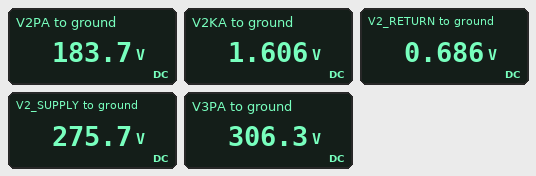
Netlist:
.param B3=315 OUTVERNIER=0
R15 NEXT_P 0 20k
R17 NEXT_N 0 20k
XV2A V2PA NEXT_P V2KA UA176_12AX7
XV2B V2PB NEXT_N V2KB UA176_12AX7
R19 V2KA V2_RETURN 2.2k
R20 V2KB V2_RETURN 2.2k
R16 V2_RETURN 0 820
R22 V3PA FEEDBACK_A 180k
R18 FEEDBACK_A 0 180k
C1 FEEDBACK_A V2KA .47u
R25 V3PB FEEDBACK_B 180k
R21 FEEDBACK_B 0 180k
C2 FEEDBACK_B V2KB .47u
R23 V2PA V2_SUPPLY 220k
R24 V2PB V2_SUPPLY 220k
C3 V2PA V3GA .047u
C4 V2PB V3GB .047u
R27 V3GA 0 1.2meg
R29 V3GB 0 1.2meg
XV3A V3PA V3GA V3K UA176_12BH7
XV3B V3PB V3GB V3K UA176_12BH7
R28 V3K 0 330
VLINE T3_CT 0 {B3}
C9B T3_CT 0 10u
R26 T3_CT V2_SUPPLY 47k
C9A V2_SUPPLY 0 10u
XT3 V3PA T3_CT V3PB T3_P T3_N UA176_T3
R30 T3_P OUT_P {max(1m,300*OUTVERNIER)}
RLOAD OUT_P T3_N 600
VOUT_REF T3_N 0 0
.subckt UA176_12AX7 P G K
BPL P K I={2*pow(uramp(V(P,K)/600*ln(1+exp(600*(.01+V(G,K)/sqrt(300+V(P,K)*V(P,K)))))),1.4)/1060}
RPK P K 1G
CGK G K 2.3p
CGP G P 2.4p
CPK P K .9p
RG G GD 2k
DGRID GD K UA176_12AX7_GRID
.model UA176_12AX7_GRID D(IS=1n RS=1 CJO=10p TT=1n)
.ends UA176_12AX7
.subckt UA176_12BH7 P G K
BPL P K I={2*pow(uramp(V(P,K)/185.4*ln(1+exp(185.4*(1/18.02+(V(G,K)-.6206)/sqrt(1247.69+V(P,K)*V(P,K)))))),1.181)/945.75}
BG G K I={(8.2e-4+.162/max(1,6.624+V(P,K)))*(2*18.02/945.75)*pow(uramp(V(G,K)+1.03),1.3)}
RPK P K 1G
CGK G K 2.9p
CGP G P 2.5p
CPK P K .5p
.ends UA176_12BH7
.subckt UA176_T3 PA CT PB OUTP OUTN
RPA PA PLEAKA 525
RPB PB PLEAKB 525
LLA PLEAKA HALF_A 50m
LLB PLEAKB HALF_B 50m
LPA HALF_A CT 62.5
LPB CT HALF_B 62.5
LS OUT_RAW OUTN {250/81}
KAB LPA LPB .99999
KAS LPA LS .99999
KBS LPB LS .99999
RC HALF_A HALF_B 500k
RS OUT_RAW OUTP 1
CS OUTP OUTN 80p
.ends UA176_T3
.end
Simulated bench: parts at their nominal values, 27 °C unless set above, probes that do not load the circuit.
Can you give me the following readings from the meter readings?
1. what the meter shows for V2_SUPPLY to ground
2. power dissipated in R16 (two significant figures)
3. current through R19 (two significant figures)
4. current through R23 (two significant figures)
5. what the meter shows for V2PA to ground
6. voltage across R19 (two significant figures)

275.7 V
570 µW
420 µA
420 µA
183.7 V
920 mV
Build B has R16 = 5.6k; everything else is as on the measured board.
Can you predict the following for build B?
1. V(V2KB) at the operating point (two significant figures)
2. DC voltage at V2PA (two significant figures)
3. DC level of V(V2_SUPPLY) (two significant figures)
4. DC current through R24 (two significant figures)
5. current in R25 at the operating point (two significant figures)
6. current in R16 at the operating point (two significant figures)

2.7 V
250 V
300 V
200 µA
850 µA
400 µA
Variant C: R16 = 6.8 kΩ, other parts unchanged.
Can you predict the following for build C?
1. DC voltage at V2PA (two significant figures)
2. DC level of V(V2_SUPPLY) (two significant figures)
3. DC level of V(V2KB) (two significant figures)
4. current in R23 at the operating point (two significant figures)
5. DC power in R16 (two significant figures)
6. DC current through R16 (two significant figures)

260 V
300 V
2.8 V
180 µA
870 µW
360 µA
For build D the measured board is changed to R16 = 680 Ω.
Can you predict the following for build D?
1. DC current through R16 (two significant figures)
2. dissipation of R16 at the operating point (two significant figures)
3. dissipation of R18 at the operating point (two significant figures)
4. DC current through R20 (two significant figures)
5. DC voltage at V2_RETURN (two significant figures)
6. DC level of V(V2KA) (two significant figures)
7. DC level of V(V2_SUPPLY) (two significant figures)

870 µA
510 µW
130 mW
430 µA
590 mV
1.5 V
270 V
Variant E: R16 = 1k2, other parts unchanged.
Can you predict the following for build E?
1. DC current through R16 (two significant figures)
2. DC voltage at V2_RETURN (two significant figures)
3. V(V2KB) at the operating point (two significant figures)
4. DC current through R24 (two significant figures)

770 µA
920 mV
1.8 V
380 µA
